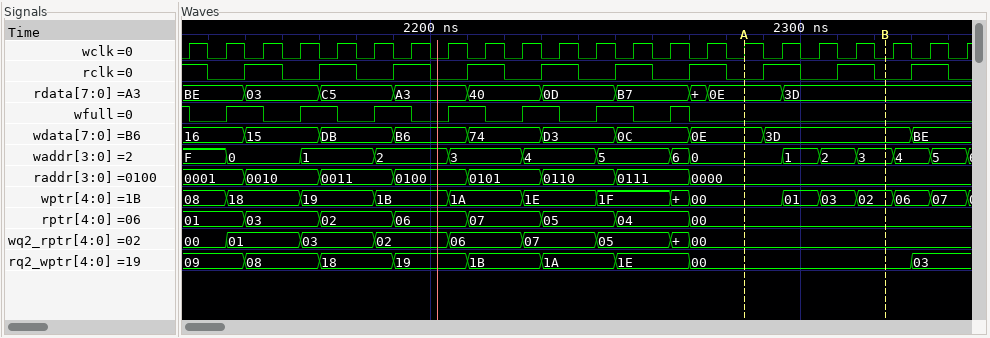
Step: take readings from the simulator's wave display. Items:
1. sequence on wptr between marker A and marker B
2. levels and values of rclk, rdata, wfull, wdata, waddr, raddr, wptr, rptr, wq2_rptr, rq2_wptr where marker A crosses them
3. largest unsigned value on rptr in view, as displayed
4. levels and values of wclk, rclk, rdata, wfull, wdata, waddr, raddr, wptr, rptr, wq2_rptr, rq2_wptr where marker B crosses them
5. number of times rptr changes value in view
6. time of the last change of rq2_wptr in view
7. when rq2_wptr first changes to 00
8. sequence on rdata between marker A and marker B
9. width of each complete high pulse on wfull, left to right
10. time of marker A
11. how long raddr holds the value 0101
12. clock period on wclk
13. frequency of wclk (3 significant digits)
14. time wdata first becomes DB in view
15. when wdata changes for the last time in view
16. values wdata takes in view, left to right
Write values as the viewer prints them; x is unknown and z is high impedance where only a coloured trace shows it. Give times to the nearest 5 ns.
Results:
00, 01, 03, 02
rclk=0, rdata=0E, wfull=0, wdata=0E, waddr=0, raddr=0000, wptr=00, rptr=00, wq2_rptr=00, rq2_wptr=00
07
wclk=0, rclk=0, rdata=3D, wfull=0, wdata=3D, waddr=3, raddr=0000, wptr=02, rptr=00, wq2_rptr=00, rq2_wptr=00
7
2330 ns
2270 ns
0E, 3D
10 ns, 10 ns, 10 ns, 10 ns, 10 ns, 10 ns, 5 ns
2285 ns
20 ns
10 ns
100 MHz
2170 ns
2330 ns
16, 15, DB, B6, 74, D3, 0C, 0E, 3D, BE
